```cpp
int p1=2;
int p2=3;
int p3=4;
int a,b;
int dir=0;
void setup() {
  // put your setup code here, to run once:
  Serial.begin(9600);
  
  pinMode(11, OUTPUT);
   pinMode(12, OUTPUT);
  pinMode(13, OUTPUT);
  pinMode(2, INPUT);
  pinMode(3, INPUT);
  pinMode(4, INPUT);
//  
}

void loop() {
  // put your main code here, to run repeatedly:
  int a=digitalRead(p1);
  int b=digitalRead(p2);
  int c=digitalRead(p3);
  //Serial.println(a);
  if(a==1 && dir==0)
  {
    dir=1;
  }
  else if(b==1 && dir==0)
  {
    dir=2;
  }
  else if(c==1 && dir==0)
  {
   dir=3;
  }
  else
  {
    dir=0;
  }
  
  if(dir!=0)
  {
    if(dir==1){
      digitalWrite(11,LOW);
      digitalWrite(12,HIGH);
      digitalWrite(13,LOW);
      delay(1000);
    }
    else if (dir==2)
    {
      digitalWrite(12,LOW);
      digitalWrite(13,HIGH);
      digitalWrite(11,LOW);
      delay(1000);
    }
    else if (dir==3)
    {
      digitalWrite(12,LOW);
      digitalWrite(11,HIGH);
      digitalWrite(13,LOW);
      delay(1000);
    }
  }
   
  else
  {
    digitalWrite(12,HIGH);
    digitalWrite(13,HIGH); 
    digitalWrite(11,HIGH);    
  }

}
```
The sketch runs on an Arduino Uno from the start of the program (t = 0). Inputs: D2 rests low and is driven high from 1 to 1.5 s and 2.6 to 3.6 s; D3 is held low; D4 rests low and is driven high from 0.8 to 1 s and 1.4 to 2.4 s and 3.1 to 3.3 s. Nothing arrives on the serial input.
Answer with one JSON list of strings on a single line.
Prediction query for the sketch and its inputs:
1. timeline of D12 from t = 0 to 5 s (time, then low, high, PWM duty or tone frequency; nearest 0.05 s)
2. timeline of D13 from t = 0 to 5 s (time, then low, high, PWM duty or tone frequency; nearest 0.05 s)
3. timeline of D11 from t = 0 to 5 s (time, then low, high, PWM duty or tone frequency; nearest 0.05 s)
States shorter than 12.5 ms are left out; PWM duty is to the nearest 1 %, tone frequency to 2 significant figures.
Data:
["0 s high; 0.8 s low; 2.8 s high", "0 s high; 0.8 s low; 3.8 s high", "0 s high; 2.8 s low; 3.8 s high"]
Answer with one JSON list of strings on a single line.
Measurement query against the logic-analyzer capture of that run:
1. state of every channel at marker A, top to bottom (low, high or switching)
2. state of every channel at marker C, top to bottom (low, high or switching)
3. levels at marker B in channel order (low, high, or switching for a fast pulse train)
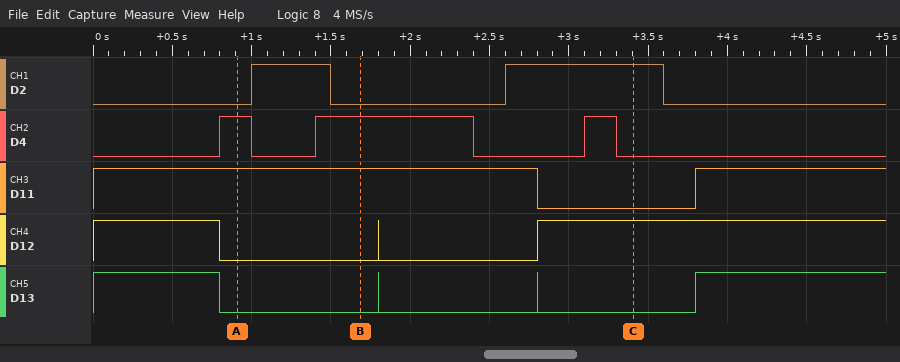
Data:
["D2 low, D4 high, D11 high, D12 low, D13 low", "D2 high, D4 low, D11 low, D12 high, D13 low", "D2 low, D4 high, D11 high, D12 low, D13 low"]
